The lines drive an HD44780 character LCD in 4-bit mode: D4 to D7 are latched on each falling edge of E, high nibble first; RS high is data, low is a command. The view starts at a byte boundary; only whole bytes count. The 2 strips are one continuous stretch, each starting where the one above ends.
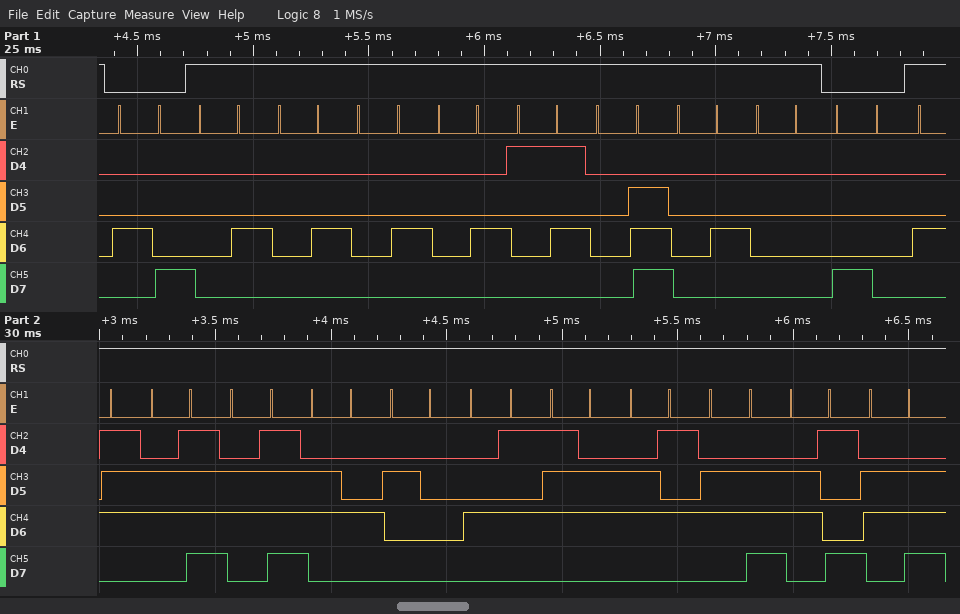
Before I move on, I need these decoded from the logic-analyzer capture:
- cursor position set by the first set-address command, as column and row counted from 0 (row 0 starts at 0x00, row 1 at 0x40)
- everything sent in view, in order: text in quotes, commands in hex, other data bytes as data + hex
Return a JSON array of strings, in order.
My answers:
["column 0, row 0", "0x48 data 04 04 04 04 15 0E 04 00 0x80 \"Good Evenin\""]
